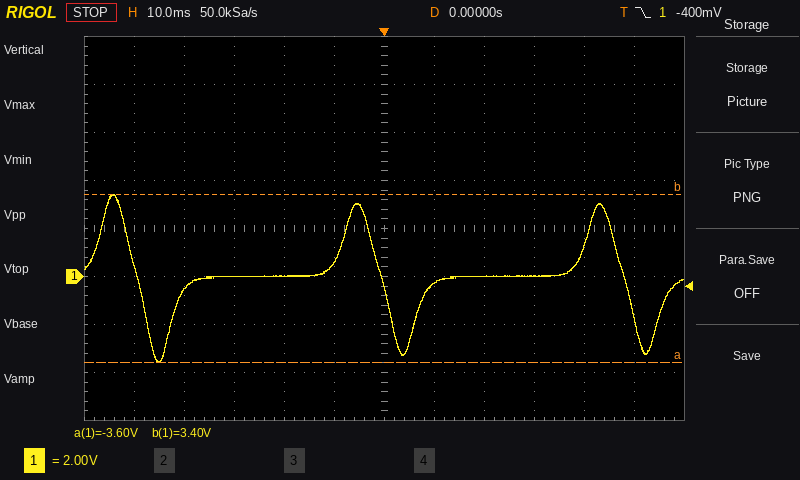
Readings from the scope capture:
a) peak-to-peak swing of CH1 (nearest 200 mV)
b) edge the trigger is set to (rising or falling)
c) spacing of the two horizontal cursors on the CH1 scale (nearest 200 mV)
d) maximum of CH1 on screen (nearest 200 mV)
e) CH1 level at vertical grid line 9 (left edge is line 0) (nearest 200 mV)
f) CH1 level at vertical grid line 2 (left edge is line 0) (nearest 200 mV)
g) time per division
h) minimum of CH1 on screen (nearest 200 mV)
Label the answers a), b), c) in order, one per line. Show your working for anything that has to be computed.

a) 3.4 V − (-3.6 V) = 7.0 V
b) falling
c) 7.0 V
d) 3.4 V
e) 0.0 V
f) -600 mV
g) 10 ms
h) -3.6 V
